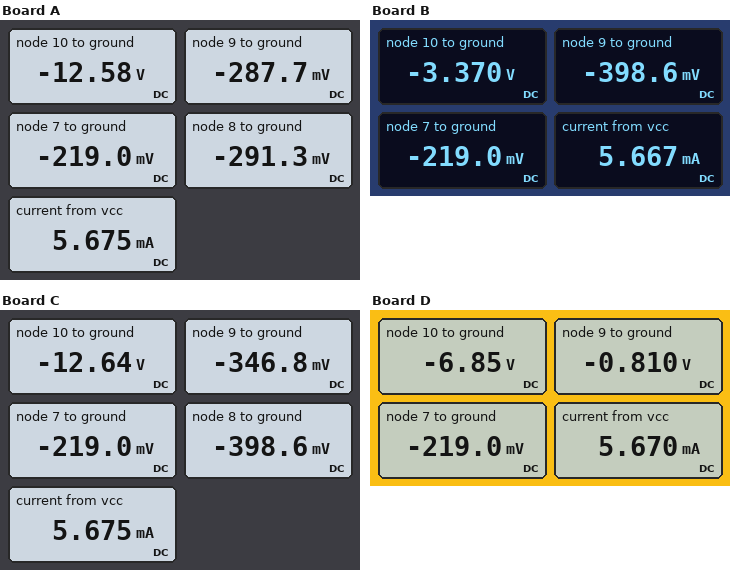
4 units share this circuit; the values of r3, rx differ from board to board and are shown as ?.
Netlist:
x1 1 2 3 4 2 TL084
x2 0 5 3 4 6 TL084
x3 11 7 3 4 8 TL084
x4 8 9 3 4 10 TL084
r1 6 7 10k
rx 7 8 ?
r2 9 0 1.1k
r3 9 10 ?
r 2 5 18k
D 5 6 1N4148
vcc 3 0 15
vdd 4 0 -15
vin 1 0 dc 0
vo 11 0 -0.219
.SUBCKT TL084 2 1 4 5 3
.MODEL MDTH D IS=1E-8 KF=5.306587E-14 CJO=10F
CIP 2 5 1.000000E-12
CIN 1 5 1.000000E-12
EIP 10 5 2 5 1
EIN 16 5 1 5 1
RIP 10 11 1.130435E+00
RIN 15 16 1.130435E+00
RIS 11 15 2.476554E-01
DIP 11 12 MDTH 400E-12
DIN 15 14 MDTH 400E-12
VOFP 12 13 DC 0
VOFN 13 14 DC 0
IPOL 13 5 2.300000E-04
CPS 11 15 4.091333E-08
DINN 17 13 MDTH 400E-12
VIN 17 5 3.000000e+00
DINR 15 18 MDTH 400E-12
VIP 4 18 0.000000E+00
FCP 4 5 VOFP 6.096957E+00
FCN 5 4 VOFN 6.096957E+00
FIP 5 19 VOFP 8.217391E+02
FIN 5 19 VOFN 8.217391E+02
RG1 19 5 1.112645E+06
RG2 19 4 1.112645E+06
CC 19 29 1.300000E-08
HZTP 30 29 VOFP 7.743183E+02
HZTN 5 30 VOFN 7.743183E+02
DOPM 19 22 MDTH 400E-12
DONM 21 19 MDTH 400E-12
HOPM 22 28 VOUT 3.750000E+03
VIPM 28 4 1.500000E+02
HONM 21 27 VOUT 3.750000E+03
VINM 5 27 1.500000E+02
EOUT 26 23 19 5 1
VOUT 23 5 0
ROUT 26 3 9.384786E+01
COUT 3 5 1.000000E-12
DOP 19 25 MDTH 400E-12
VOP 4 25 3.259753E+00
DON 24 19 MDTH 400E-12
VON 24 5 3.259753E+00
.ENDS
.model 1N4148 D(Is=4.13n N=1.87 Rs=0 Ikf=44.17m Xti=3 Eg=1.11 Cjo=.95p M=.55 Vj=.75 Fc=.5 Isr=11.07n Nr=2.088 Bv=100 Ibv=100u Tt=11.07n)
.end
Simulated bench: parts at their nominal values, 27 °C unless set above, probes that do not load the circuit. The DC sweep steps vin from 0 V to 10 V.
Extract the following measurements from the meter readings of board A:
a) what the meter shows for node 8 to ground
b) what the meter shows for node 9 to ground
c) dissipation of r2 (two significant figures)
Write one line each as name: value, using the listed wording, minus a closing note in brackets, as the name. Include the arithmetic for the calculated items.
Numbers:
what the meter shows for node 8 to ground: -291.3 mV
what the meter shows for node 9 to ground: -287.7 mV
dissipation of r2: (0 V - (-287.7 mV))^2 / 1.1 kΩ = 75 µW
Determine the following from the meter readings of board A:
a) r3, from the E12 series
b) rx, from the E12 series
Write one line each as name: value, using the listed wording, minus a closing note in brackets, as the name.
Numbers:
r3, from the E12 series: 47 kΩ
rx, from the E12 series: 3.3 kΩ
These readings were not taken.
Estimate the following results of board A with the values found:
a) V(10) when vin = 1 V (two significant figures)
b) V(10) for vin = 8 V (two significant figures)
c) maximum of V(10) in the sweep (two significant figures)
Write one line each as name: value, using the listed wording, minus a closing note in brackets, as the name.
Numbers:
V(10) when vin = 1 V: -6.4 V
V(10) for vin = 8 V: -4.8 V
maximum of V(10) in the sweep: -4.6 V
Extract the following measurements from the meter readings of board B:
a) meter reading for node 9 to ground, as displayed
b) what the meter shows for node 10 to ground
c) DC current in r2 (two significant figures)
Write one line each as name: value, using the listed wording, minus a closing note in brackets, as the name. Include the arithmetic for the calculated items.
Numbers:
meter reading for node 9 to ground, as displayed: -398.6 mV
what the meter shows for node 10 to ground: -3.370 V
DC current in r2: (0 V - (-398.6 mV)) / 1.1 kΩ = 360 µA
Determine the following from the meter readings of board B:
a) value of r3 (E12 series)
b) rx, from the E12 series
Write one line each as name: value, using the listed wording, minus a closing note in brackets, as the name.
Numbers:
value of r3: 8.2 kΩ
rx, from the E12 series: 8.2 kΩ
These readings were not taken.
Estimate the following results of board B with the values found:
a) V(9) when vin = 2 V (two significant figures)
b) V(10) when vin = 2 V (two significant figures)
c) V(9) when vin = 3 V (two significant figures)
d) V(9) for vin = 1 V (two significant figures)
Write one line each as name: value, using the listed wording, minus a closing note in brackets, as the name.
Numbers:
V(9) when vin = 2 V: -9.7 mV
V(10) when vin = 2 V: -82 mV
V(9) when vin = 3 V: 8.1 mV
V(9) for vin = 1 V: -40 mV
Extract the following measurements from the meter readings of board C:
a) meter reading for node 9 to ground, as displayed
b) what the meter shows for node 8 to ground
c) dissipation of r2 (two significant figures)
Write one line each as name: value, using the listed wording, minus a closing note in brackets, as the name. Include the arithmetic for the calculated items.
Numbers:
meter reading for node 9 to ground, as displayed: -346.8 mV
what the meter shows for node 8 to ground: -398.6 mV
dissipation of r2: (0 V - (-346.8 mV))^2 / 1.1 kΩ = 110 µW
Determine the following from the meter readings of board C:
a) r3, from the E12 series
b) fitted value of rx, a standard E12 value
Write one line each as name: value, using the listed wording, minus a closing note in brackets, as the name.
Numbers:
r3, from the E12 series: 39 kΩ
fitted value of rx, a standard E12 value: 8.2 kΩ
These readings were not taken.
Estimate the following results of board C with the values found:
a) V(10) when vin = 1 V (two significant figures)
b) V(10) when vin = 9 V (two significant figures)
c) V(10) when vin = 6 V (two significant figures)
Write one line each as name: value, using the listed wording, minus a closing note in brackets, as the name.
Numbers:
V(10) when vin = 1 V: -1.5 V
V(10) when vin = 9 V: 2.1 V
V(10) when vin = 6 V: 1.4 V
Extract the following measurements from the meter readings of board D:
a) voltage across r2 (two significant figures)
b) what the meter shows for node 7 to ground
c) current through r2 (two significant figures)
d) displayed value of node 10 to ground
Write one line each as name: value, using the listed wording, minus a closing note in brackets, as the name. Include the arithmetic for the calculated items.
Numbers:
voltage across r2: 0 V - (-810 mV) = 810 mV
what the meter shows for node 7 to ground: -219.0 mV
current through r2: (0 V - (-810 mV)) / 1.1 kΩ = 740 µA
displayed value of node 10 to ground: -6.85 V
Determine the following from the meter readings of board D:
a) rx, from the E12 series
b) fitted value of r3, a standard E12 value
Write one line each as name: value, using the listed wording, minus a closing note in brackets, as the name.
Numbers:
rx, from the E12 series: 27 kΩ
fitted value of r3, a standard E12 value: 8.2 kΩ
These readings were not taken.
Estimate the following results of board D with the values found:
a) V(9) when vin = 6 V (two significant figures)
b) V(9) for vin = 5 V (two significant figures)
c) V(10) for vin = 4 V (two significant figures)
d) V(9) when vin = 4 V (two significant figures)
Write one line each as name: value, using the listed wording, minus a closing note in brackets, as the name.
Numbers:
V(9) when vin = 6 V: 630 mV
V(9) for vin = 5 V: 600 mV
V(10) for vin = 4 V: 4.8 V
V(9) when vin = 4 V: 570 mV
